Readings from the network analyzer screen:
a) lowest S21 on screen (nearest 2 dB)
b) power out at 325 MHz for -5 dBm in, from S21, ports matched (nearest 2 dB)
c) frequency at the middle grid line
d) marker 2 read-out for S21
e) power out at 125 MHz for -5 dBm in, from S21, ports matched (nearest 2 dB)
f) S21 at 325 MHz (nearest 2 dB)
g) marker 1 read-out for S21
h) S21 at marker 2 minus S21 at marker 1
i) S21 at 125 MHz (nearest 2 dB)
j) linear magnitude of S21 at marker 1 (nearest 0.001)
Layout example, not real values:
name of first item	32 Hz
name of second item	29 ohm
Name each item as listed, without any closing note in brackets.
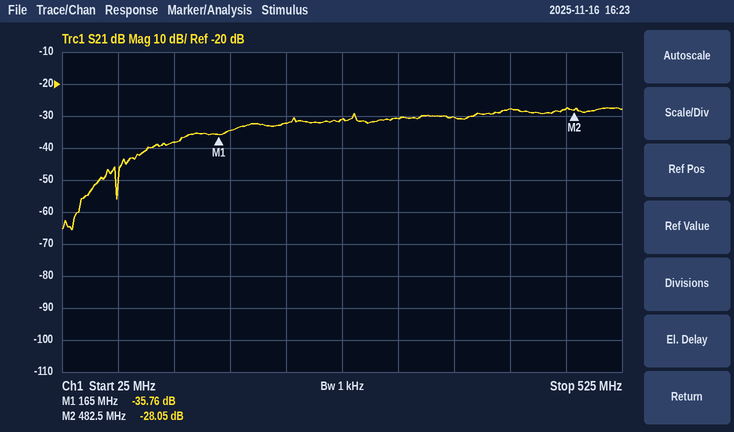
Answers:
lowest S21 on screen	-66 dB
power out at 325 MHz for -5 dBm in, from S21, ports matched	-36 dBm
frequency at the middle grid line	275 MHz
marker 2 read-out for S21	-28.05 dB
power out at 125 MHz for -5 dBm in, from S21, ports matched	-44 dBm
S21 at 325 MHz	-30 dB
marker 1 read-out for S21	-35.76 dB
S21 at marker 2 minus S21 at marker 1	7.71 dB
S21 at 125 MHz	-38 dB
linear magnitude of S21 at marker 1	0.016
